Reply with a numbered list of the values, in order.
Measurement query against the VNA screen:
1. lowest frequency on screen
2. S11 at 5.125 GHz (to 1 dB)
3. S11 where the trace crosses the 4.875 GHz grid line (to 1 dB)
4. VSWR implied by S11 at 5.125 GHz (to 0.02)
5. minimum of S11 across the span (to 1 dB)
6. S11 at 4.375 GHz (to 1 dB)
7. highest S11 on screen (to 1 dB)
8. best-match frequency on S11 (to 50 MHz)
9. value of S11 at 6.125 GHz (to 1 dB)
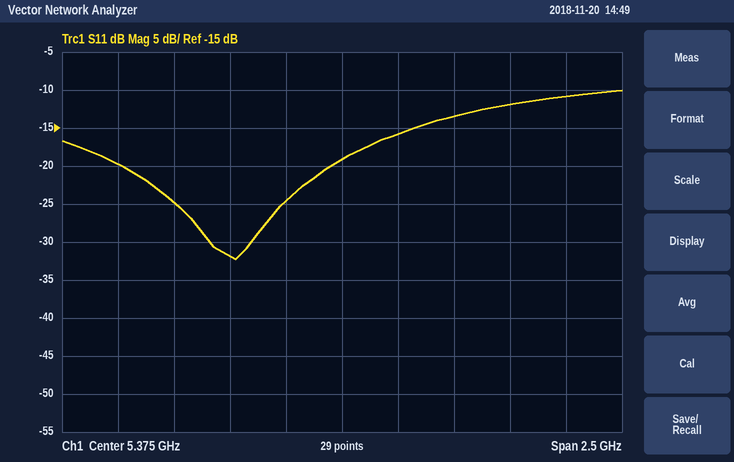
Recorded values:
1. 4.125 GHz
2. -25 dB
3. -32 dB
4. 1.12
5. -32 dB
6. -20 dB
7. -10 dB
8. 4.90 GHz
9. -12 dB
